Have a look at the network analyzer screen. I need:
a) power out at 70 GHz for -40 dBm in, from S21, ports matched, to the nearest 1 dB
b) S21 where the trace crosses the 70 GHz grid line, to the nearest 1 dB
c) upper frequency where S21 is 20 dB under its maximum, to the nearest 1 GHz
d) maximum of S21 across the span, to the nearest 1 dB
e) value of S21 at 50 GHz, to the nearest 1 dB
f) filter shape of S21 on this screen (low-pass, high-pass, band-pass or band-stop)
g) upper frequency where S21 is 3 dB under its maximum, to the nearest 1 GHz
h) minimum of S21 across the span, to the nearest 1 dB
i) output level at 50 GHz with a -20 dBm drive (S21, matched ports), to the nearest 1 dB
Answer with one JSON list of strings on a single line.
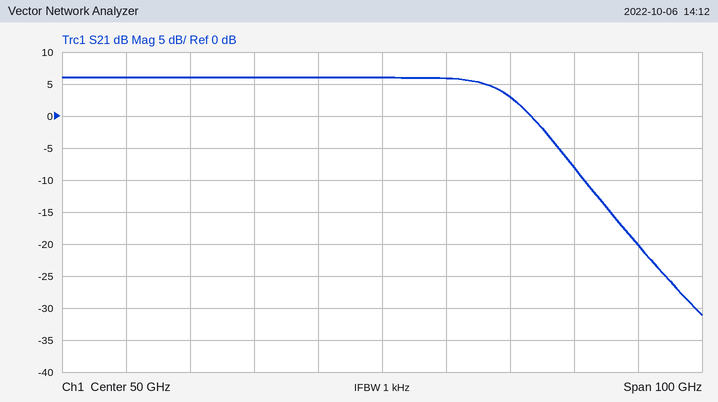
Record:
["-37 dBm", "3 dB", "85 GHz", "6 dB", "6 dB", "low-pass", "70 GHz", "-31 dB", "-14 dBm"]
